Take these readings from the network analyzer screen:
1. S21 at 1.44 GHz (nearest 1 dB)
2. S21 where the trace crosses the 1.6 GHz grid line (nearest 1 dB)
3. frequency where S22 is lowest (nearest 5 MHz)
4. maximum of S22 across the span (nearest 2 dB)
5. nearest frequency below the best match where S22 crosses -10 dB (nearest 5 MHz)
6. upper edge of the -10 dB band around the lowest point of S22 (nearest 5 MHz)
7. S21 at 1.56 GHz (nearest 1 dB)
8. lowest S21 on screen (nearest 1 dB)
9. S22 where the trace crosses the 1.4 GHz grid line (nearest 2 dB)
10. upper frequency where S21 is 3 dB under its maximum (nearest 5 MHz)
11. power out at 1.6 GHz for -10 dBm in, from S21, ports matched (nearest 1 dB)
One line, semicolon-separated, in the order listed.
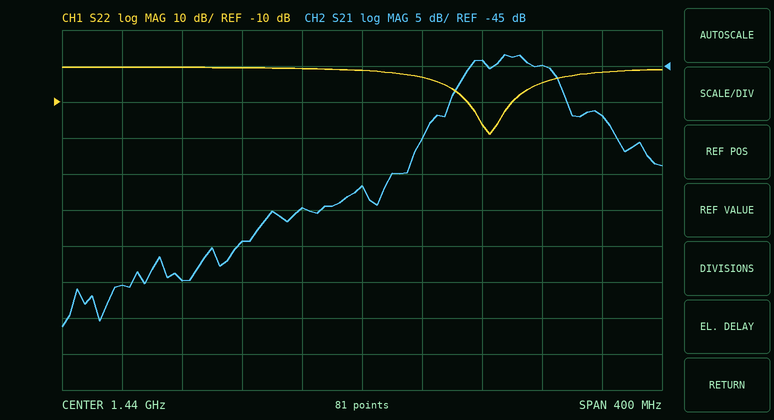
-62 dB; -52 dB; 1.525 GHz; 0 dB; 1.510 GHz; 1.540 GHz; -45 dB; -81 dB; 0 dB; 1.570 GHz; -62 dBm
